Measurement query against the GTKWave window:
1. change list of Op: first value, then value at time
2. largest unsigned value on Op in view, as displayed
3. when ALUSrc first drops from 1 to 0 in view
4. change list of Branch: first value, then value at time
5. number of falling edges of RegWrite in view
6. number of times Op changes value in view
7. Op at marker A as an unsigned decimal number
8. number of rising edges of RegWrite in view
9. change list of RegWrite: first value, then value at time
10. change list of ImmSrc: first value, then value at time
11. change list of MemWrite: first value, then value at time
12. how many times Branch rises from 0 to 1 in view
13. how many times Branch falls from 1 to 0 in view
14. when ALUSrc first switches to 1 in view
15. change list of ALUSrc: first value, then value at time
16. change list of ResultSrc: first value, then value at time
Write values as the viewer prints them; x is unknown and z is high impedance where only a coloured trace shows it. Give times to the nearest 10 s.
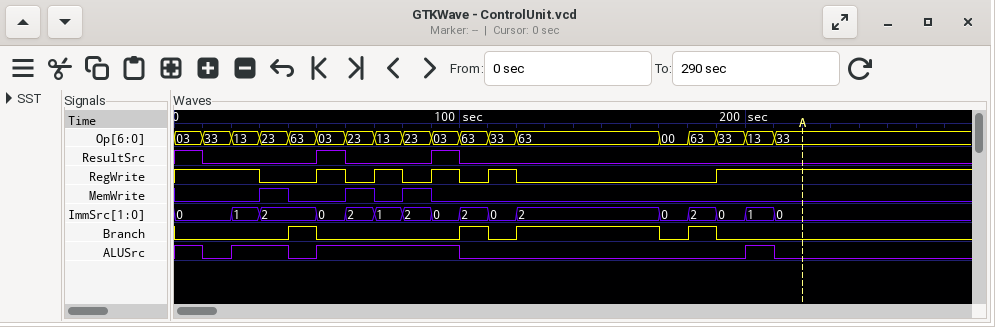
03, 33 at 10 s, 13 at 20 s, 23 at 30 s, 63 at 40 s, 03 at 50 s, 23 at 60 s, 13 at 70 s, 23 at 80 s, 03 at 90 s, 63 at 100 s, 33 at 110 s, 63 at 120 s, 00 at 170 s, 63 at 180 s, 33 at 190 s, 13 at 200 s, 33 at 210 s
63
10 s
0, 1 at 40 s, 0 at 50 s, 1 at 100 s, 0 at 110 s, 1 at 120 s, 0 at 170 s, 1 at 180 s, 0 at 190 s
5
17
51
5
1, 0 at 30 s, 1 at 50 s, 0 at 60 s, 1 at 70 s, 0 at 80 s, 1 at 90 s, 0 at 100 s, 1 at 110 s, 0 at 120 s, 1 at 190 s
0, 1 at 20 s, 2 at 30 s, 0 at 50 s, 2 at 60 s, 1 at 70 s, 2 at 80 s, 0 at 90 s, 2 at 100 s, 0 at 110 s, 2 at 120 s, 0 at 170 s, 2 at 180 s, 0 at 190 s, 1 at 200 s, 0 at 210 s
0, 1 at 30 s, 0 at 40 s, 1 at 60 s, 0 at 70 s, 1 at 80 s, 0 at 90 s
4
4
20 s
1, 0 at 10 s, 1 at 20 s, 0 at 40 s, 1 at 50 s, 0 at 100 s, 1 at 200 s, 0 at 210 s
1, 0 at 10 s, 1 at 50 s, 0 at 60 s, 1 at 90 s, 0 at 100 s
